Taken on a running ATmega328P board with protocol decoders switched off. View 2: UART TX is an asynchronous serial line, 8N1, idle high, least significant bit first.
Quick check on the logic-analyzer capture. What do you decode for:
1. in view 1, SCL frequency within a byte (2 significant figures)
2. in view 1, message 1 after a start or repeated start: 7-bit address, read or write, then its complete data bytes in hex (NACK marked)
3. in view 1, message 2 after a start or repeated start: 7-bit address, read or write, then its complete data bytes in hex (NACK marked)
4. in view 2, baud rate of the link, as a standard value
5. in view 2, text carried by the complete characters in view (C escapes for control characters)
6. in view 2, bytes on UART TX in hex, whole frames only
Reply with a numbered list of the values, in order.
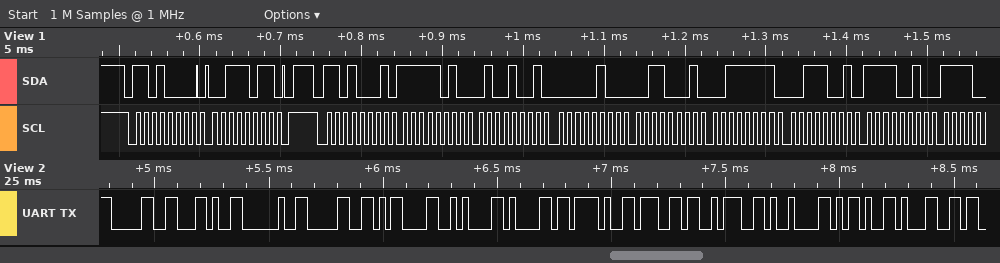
1. 100 kHz
2. 0x68 write: 3B
3. 0x68 read: FA 49 04 31 3F 39 F2
4. 38400 baud
5. "0, 0\r\na/g:\t-1"
6. 0x30 0x2C 0x20 0x30 0x0D 0x0A 0x61 0x2F 0x67 0x3A 0x09 0x2D 0x31
